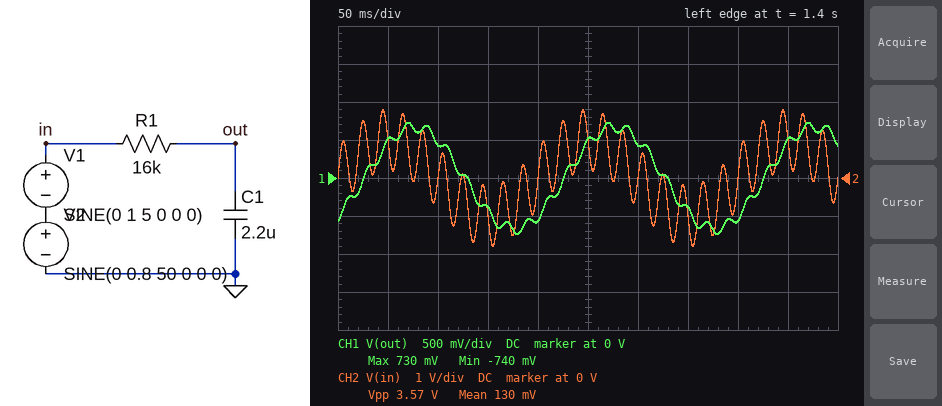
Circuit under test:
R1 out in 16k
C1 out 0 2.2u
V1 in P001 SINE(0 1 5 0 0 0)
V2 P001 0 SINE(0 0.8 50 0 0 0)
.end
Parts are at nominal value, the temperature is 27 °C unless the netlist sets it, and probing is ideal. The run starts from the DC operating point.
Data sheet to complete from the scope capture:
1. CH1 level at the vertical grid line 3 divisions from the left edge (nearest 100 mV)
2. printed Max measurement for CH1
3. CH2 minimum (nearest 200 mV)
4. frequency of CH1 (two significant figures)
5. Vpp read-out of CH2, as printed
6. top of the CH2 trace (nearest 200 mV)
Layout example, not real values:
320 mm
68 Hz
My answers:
-400 mV
730 mV
-1.8 V
5.0 Hz
3.57 V
1.8 V
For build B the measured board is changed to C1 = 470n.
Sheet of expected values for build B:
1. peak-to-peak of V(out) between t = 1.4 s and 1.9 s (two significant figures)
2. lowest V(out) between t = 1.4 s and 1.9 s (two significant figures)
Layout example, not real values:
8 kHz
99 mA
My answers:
2.5 V
-1.3 V
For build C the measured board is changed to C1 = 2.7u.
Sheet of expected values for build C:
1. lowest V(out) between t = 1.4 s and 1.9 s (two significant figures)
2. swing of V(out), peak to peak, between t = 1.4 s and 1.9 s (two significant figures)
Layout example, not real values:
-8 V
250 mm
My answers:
-650 mV
1.3 V
